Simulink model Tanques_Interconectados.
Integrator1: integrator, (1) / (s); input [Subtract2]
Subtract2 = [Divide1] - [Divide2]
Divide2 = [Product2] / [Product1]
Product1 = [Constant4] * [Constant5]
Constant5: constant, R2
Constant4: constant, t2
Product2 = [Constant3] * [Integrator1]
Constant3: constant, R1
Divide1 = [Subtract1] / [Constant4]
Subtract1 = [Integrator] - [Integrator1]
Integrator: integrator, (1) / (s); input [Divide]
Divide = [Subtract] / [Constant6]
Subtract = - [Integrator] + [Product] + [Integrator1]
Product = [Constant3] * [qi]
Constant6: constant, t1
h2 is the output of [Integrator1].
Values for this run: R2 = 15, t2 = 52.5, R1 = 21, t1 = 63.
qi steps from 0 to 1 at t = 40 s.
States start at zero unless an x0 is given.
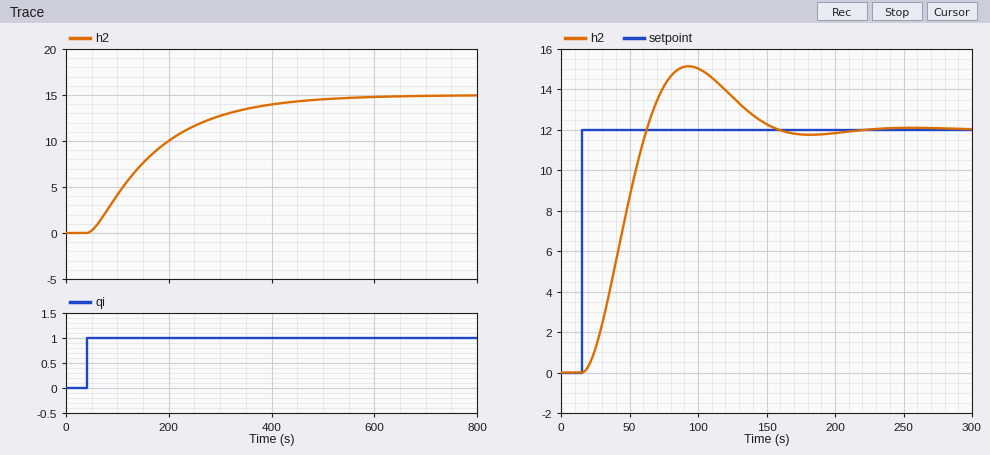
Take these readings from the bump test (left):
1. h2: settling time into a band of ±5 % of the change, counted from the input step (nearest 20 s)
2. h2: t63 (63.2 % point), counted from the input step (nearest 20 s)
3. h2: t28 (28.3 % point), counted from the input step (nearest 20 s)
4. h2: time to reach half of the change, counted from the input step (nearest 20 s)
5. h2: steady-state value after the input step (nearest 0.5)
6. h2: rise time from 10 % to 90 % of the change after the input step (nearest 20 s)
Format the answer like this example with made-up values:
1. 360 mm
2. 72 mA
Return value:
1. 400 s
2. 140 s
3. 60 s
4. 100 s
5. 15.0
6. 280 s
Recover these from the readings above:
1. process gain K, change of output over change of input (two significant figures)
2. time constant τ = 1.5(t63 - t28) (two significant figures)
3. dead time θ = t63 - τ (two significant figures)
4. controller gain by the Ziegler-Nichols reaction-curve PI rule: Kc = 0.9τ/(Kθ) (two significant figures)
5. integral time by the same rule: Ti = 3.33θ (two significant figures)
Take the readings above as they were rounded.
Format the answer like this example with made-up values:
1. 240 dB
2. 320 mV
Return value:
1. 15
2. 120 s
3. 20 s
4. 0.36
5. 67 s
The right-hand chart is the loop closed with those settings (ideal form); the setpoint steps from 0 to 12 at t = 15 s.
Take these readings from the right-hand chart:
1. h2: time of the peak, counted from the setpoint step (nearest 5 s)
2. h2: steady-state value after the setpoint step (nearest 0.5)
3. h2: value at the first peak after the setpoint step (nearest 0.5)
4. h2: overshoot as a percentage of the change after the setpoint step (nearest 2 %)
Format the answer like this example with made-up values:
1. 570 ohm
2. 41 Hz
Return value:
1. 80 s
2. 12.0
3. 15.0
4. 26 %
